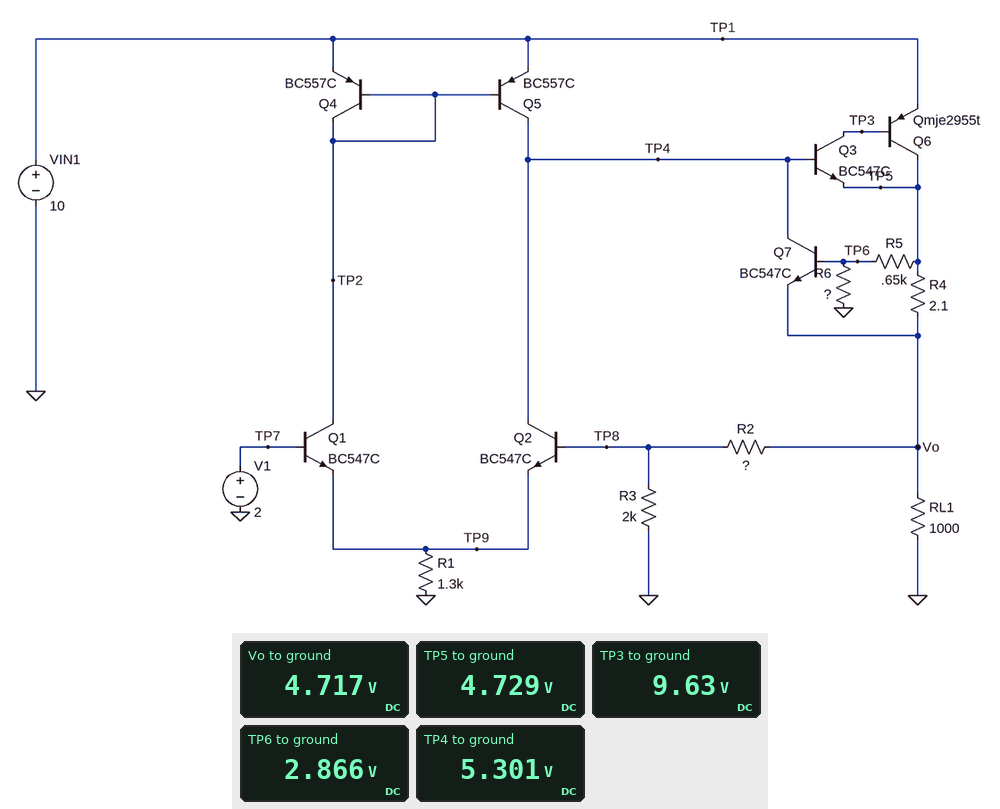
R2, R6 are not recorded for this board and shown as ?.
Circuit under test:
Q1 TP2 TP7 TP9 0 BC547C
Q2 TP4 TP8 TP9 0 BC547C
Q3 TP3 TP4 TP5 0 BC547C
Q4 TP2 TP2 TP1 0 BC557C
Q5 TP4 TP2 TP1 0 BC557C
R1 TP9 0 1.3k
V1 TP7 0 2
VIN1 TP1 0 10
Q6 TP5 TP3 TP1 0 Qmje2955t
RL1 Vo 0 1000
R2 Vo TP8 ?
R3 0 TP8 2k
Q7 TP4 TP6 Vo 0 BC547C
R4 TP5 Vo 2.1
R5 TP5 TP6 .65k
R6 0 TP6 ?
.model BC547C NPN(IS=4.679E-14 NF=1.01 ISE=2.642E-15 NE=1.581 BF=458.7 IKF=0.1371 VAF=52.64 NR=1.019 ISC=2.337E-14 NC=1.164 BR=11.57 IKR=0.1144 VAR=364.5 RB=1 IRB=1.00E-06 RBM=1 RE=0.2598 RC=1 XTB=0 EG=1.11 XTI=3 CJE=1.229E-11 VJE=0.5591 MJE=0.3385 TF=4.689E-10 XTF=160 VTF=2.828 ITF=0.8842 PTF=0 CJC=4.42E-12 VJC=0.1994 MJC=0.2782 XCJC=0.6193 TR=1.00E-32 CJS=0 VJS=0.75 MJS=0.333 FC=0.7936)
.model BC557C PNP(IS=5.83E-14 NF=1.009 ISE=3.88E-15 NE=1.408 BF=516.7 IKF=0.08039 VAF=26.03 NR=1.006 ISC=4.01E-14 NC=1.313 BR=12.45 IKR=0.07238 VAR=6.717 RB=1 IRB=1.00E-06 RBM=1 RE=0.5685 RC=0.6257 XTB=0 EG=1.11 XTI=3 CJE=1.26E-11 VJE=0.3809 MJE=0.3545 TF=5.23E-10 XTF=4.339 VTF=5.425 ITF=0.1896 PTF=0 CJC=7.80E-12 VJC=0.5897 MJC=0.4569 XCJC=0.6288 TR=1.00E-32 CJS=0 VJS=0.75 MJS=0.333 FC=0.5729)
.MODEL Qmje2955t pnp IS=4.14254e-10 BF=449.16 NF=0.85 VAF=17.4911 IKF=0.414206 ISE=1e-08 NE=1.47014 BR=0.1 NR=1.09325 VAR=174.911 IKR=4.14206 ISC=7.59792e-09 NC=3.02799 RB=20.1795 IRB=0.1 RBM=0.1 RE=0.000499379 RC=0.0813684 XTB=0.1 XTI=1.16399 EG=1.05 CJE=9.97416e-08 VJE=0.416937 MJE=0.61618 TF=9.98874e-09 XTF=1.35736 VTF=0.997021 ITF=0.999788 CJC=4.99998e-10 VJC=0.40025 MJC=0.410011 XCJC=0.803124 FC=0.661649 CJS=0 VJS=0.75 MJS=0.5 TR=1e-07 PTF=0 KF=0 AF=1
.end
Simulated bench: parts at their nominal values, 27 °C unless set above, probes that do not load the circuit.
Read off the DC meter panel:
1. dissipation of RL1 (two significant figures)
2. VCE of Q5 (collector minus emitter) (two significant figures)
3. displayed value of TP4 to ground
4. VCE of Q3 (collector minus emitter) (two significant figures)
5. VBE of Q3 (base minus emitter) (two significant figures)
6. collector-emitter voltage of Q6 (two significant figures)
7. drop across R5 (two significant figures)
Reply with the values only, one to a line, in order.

22 mW
-4.7 V
5.301 V
4.9 V
570 mV
-5.3 V
1.9 V
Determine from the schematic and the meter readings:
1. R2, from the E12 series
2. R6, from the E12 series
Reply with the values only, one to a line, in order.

2.7 kΩ
1 kΩ
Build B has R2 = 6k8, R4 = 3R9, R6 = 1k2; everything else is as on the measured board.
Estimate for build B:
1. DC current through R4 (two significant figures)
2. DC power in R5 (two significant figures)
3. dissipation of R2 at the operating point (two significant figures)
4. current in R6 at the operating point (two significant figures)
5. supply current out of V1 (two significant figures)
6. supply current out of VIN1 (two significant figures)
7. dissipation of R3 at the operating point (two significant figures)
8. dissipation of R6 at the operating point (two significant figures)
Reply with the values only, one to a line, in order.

9.8 mA
15 mW
6.8 mW
4.8 mA
1.0 µA
16 mA
2.0 mW
27 mW
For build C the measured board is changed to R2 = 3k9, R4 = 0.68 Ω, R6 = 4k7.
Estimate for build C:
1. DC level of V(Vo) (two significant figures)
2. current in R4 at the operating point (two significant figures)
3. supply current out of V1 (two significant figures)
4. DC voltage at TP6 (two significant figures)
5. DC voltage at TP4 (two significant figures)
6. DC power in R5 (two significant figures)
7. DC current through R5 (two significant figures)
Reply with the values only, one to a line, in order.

5.9 V
6.9 mA
980 nA
5.2 V
6.5 V
800 µW
1.1 mA
